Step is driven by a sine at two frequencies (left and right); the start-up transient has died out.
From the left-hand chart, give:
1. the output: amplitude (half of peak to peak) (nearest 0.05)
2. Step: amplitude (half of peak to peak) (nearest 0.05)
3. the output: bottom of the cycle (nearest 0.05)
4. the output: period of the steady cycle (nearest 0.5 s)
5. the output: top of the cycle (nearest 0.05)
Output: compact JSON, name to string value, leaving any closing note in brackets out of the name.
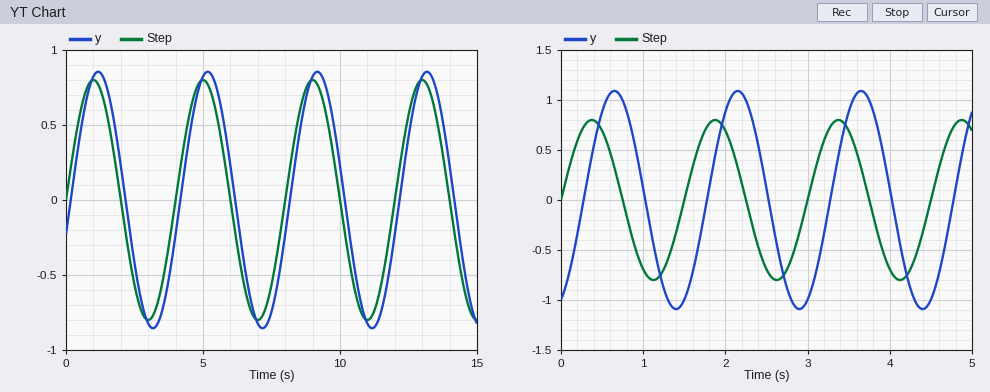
{"the output: amplitude (half of peak to peak)": "0.85", "Step: amplitude (half of peak to peak)": "0.80", "the output: bottom of the cycle": "-0.85", "the output: period of the steady cycle": "4.0 s", "the output: top of the cycle": "0.85"}
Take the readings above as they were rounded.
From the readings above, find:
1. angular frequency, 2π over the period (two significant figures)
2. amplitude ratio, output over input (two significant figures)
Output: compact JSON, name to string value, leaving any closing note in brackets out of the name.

{"angular frequency, 2π over the period": "1.6 rad/s", "amplitude ratio, output over input": "1.1"}
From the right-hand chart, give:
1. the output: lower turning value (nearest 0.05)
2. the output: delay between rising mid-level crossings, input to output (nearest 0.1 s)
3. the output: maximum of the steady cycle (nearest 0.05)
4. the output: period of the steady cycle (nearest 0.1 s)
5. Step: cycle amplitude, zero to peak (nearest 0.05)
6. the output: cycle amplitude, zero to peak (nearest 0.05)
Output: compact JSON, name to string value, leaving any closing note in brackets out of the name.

{"the output: lower turning value": "-1.10", "the output: delay between rising mid-level crossings, input to output": "0.3 s", "the output: maximum of the steady cycle": "1.10", "the output: period of the steady cycle": "1.5 s", "Step: cycle amplitude, zero to peak": "0.80", "the output: cycle amplitude, zero to peak": "1.10"}
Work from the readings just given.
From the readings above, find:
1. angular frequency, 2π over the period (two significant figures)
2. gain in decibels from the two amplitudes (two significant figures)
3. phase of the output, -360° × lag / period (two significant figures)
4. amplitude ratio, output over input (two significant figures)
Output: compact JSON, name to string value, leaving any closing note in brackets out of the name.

{"angular frequency, 2π over the period": "4.2 rad/s", "gain in decibels from the two amplitudes": "2.8 dB", "phase of the output, -360° × lag / period": "-72°", "amplitude ratio, output over input": "1.4"}
